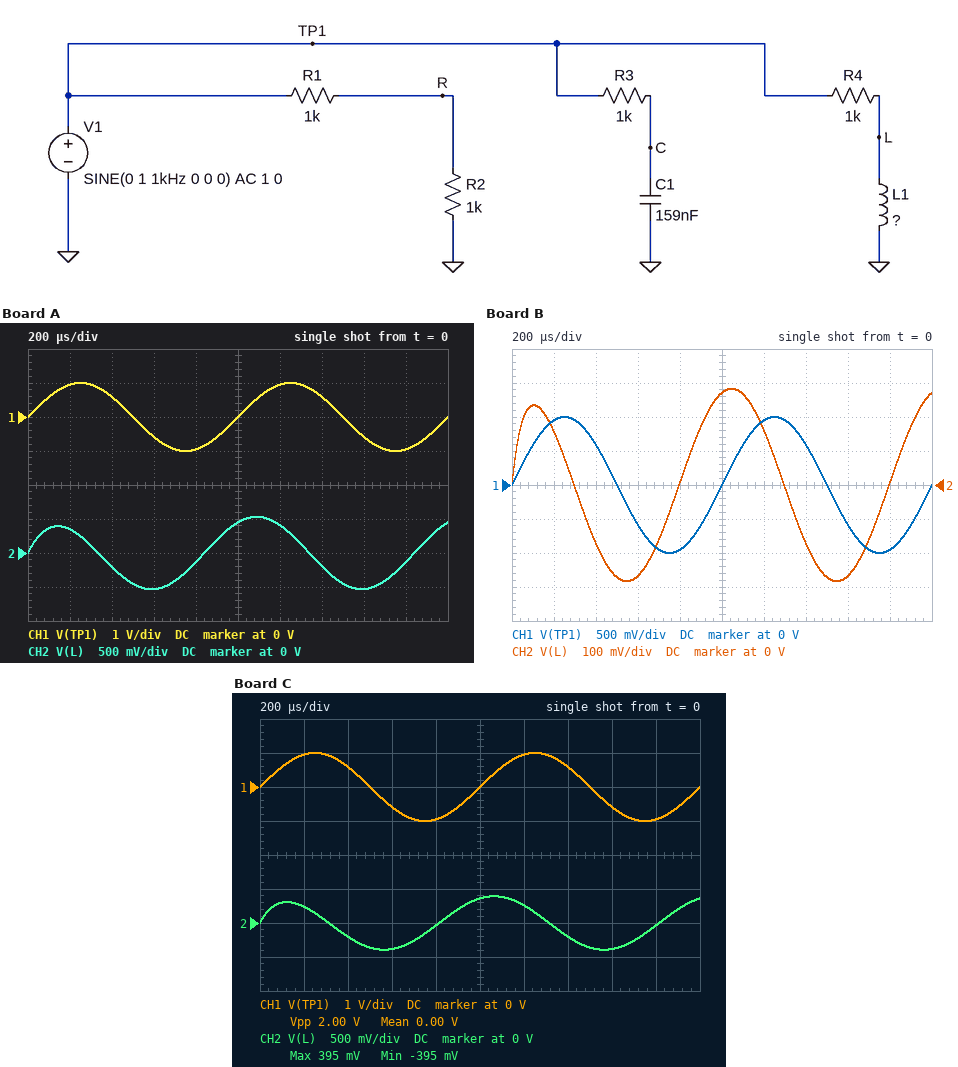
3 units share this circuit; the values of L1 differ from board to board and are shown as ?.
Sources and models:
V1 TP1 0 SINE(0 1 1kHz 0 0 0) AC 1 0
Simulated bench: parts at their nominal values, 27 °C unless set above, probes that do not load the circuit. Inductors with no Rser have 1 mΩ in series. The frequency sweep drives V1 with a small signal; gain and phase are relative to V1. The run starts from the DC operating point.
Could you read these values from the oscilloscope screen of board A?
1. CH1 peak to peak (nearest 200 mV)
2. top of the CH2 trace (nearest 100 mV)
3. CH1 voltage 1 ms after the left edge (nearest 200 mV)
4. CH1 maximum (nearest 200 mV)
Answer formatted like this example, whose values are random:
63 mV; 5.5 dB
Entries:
2.0 V; 500 mV; 0 V; 1.0 V
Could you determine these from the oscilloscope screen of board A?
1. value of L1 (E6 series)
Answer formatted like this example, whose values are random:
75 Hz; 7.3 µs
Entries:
100 mH
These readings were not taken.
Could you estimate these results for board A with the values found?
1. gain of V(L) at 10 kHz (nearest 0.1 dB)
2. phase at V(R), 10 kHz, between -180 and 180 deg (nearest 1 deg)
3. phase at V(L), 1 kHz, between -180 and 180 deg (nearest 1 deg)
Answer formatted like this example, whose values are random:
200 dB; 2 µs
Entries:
-0.1 dB; 0 deg; 58 deg
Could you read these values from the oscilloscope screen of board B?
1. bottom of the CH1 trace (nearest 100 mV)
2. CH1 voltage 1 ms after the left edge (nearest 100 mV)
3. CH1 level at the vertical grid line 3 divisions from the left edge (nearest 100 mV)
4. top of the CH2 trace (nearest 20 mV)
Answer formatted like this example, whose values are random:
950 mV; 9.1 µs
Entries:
-1.0 V; 0 V; -600 mV; 280 mV
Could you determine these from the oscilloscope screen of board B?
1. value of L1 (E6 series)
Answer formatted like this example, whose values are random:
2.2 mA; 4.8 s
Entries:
47 mH
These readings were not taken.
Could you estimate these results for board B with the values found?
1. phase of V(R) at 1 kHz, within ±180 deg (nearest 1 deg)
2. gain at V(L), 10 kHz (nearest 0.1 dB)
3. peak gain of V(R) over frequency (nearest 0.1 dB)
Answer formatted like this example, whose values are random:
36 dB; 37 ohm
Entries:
0 deg; -0.5 dB; -6.0 dB
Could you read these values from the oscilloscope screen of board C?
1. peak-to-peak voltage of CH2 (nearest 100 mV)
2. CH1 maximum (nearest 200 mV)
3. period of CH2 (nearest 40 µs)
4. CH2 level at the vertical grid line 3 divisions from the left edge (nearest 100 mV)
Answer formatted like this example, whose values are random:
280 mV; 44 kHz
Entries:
800 mV; 1.0 V; 1.00 ms; -400 mV
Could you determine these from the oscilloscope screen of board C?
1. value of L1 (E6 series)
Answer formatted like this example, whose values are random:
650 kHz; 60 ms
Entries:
68 mH
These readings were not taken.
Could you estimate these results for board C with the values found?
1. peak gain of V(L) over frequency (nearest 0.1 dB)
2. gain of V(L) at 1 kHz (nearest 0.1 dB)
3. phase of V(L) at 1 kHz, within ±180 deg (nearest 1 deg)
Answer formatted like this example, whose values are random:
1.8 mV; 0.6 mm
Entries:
0 dB; -8.1 dB; 67 deg
